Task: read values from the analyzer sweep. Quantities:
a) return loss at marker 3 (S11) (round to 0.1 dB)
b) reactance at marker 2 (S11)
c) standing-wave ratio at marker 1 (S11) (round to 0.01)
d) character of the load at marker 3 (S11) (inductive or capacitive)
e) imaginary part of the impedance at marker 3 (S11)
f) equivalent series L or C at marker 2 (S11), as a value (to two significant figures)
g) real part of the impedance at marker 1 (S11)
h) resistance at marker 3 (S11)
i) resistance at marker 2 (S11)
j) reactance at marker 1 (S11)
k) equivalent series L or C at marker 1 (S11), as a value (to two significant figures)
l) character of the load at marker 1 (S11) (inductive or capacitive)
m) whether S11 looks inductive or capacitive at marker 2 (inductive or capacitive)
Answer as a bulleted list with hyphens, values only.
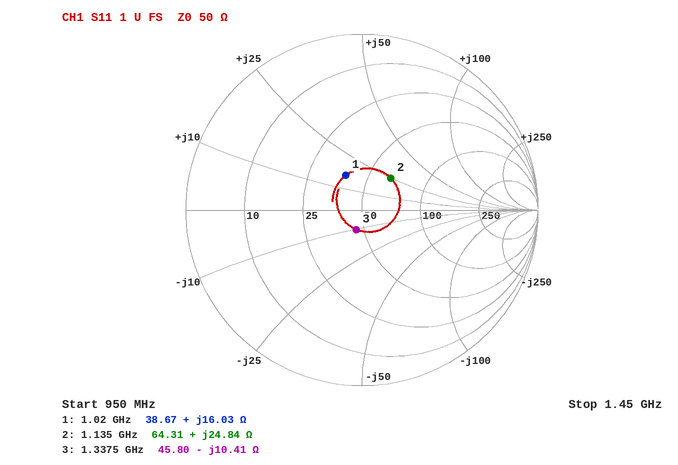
- 18.7 dB
- +24.84 Ω
- 1.56
- capacitive
- -10.41 Ω
- 3.5 nH
- 38.67 Ω
- 45.80 Ω
- 64.31 Ω
- +16.03 Ω
- 2.5 nH
- inductive
- inductive
